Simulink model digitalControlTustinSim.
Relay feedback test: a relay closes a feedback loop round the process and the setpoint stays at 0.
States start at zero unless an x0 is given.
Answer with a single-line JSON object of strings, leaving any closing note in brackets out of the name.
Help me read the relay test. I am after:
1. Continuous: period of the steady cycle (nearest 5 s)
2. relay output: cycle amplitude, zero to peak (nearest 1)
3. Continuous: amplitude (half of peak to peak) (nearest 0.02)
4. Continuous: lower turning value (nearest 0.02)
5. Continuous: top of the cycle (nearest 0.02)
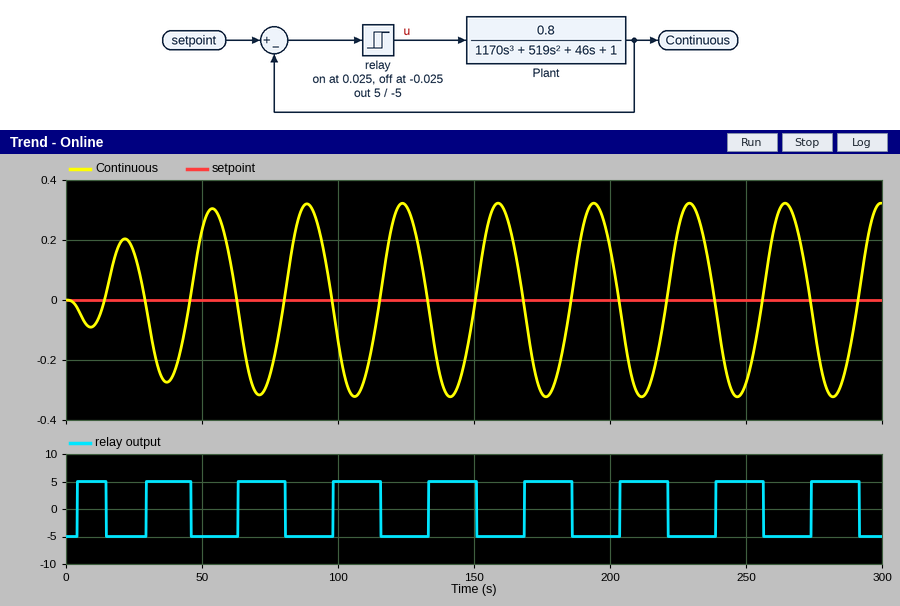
{"Continuous: period of the steady cycle": "35 s", "relay output: cycle amplitude, zero to peak": "5", "Continuous: amplitude (half of peak to peak)": "0.32", "Continuous: lower turning value": "-0.32", "Continuous: top of the cycle": "0.32"}
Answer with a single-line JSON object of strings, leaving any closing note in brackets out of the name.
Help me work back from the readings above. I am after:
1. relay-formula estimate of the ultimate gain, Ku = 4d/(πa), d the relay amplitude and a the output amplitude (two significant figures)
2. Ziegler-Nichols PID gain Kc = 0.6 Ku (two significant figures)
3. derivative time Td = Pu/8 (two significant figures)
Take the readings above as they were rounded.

{"relay-formula estimate of the ultimate gain, Ku = 4d/(πa), d the relay amplitude and a the output amplitude": "20", "Ziegler-Nichols PID gain Kc = 0.6 Ku": "12", "derivative time Td = Pu/8": "4.4 s"}
